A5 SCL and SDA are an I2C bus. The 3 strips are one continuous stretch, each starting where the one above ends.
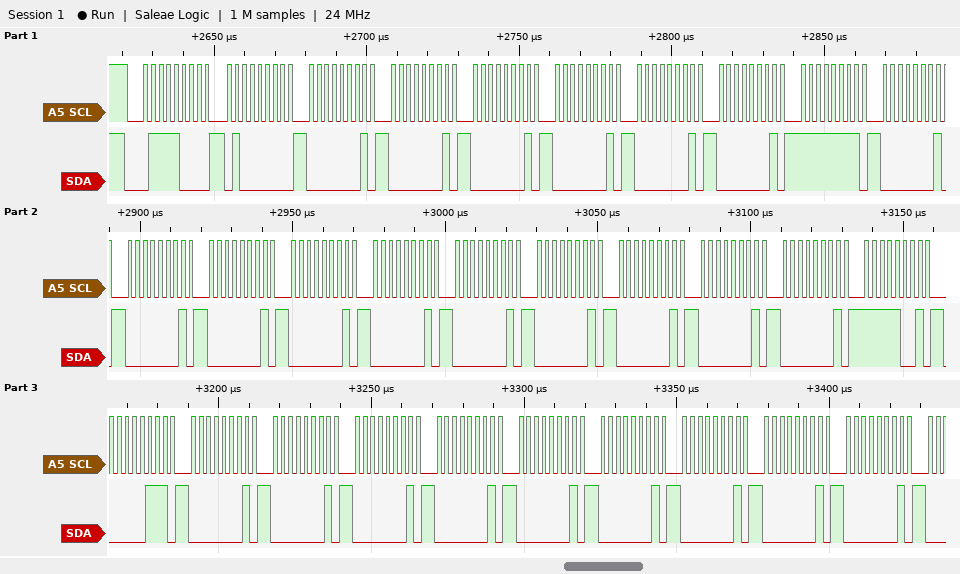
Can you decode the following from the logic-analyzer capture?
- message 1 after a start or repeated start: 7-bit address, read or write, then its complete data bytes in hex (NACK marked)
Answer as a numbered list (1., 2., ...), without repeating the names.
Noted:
1. 0x3C write: 40 01 01 01 01 01 01 FF 01 01 01 01 01 01 01 01 01 01 F9 07 01 01 01 01 01 01 01 01 01
